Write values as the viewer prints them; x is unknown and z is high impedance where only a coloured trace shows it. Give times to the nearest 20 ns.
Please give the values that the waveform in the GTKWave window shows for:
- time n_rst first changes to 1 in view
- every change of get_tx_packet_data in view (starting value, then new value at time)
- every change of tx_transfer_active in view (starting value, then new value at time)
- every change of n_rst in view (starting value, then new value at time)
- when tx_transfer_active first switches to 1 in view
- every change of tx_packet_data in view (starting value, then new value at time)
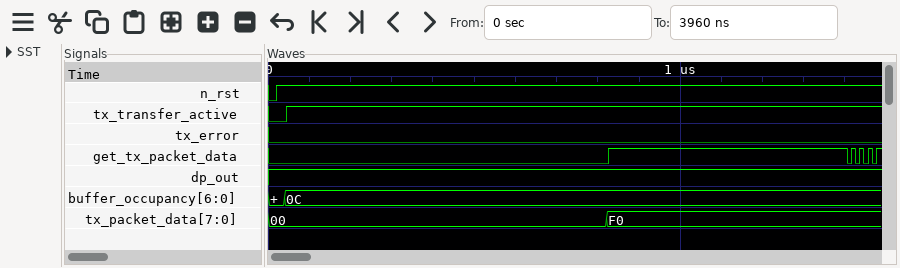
20 ns
0, 1 at 820 ns, 0 at 1400 ns, 1 at 1420 ns, 0 at 1420 ns, 1 at 1440 ns, 0 at 1440 ns, 1 at 1460 ns, 0 at 1460 ns, 1 at 1480 ns
0, 1 at 40 ns
0, 1 at 20 ns
40 ns
00, F0 at 820 ns
